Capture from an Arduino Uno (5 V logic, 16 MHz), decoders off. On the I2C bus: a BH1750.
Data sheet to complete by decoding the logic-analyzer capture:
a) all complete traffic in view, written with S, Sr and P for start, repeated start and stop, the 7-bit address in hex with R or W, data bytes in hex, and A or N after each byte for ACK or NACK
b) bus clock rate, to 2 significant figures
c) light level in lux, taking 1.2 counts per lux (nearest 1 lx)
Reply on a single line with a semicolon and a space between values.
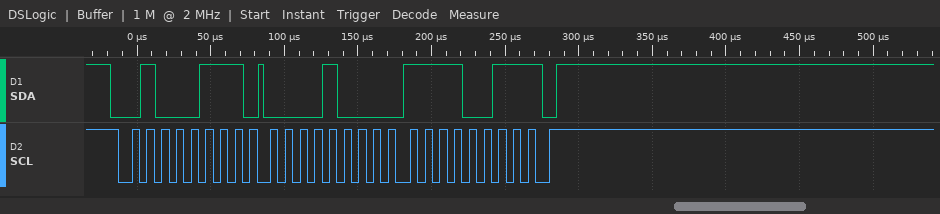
S 23R A 08 A F3 N P; 100 kHz; 1909 lx
